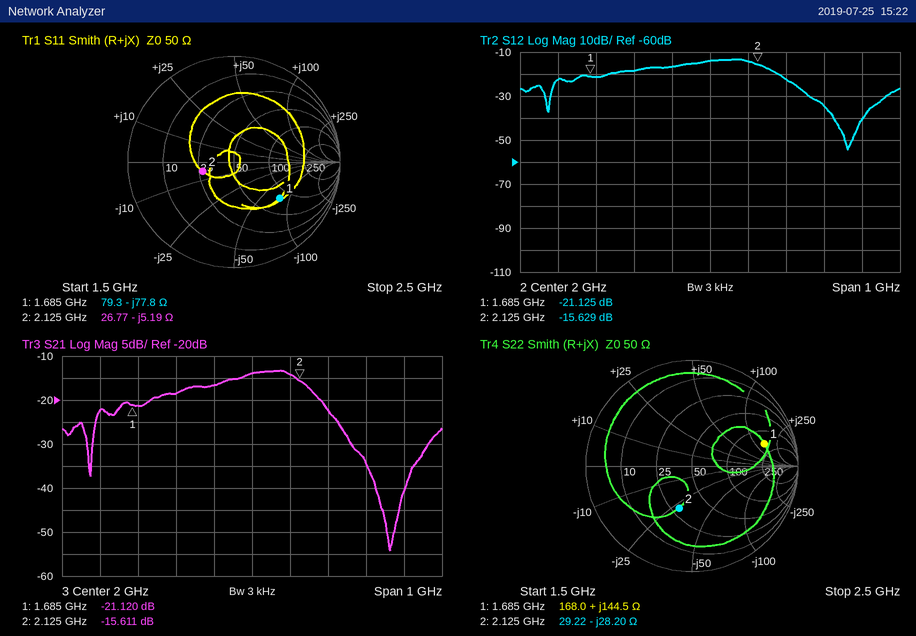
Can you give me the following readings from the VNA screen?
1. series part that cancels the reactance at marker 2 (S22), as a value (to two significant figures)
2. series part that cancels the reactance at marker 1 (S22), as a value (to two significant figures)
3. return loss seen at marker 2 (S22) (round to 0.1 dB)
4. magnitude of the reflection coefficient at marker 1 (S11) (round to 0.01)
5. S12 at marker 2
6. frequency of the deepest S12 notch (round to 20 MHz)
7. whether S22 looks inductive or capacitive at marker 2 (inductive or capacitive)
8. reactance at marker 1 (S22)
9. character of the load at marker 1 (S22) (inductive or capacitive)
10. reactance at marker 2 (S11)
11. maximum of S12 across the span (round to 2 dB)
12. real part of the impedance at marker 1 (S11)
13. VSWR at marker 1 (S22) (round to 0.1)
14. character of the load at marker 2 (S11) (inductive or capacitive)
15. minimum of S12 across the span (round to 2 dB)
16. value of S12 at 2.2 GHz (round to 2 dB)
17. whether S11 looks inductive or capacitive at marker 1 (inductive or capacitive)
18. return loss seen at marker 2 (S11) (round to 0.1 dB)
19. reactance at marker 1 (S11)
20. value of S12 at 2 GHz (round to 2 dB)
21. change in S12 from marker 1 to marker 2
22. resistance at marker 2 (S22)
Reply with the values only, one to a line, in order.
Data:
2.1 nH
650 fF
7.6 dB
0.55
-15.629 dB
2.36 GHz
capacitive
+144.5 Ω
inductive
-5.19 Ω
-14 dB
79.3 Ω
6.0
capacitive
-54 dB
-22 dB
capacitive
10.2 dB
-77.8 Ω
-14 dB
5.496 dB
29.22 Ω
